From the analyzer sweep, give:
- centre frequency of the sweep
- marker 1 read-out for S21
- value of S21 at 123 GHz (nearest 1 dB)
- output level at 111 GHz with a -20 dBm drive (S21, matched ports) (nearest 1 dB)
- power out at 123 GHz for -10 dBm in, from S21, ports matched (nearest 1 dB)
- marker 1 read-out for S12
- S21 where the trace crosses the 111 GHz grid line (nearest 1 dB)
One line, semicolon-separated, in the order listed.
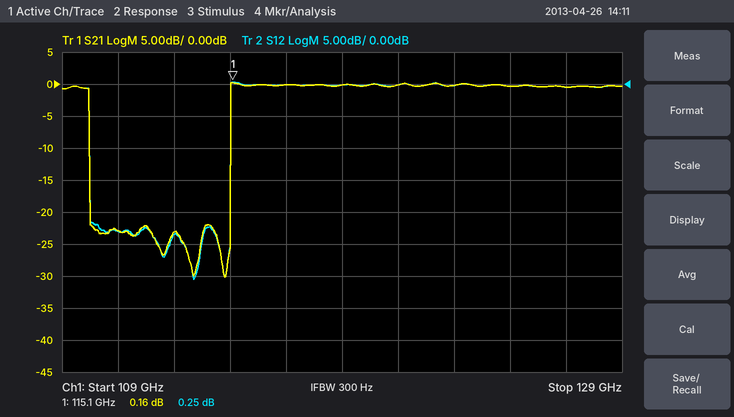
119 GHz; 0.16 dB; 0 dB; -43 dBm; -10 dBm; 0.25 dB; -23 dB
